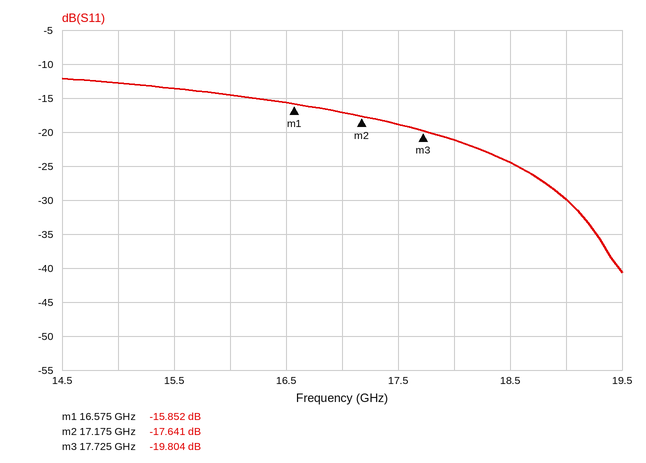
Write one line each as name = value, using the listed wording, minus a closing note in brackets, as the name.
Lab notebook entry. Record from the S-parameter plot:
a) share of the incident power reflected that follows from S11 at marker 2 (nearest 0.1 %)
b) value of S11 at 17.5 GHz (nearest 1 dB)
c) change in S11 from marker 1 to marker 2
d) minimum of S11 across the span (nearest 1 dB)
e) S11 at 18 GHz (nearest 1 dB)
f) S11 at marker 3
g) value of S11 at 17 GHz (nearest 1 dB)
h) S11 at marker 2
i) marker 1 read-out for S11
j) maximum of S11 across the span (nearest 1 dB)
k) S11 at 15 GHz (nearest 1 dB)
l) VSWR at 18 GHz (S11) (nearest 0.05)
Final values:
share of the incident power reflected that follows from S11 at marker 2 = 1.7 %
value of S11 at 17.5 GHz = -19 dB
change in S11 from marker 1 to marker 2 = -1.789 dB
minimum of S11 across the span = -41 dB
S11 at 18 GHz = -21 dB
S11 at marker 3 = -19.804 dB
value of S11 at 17 GHz = -17 dB
S11 at marker 2 = -17.641 dB
marker 1 read-out for S11 = -15.852 dB
maximum of S11 across the span = -12 dB
S11 at 15 GHz = -13 dB
VSWR at 18 GHz (S11) = 1.20
